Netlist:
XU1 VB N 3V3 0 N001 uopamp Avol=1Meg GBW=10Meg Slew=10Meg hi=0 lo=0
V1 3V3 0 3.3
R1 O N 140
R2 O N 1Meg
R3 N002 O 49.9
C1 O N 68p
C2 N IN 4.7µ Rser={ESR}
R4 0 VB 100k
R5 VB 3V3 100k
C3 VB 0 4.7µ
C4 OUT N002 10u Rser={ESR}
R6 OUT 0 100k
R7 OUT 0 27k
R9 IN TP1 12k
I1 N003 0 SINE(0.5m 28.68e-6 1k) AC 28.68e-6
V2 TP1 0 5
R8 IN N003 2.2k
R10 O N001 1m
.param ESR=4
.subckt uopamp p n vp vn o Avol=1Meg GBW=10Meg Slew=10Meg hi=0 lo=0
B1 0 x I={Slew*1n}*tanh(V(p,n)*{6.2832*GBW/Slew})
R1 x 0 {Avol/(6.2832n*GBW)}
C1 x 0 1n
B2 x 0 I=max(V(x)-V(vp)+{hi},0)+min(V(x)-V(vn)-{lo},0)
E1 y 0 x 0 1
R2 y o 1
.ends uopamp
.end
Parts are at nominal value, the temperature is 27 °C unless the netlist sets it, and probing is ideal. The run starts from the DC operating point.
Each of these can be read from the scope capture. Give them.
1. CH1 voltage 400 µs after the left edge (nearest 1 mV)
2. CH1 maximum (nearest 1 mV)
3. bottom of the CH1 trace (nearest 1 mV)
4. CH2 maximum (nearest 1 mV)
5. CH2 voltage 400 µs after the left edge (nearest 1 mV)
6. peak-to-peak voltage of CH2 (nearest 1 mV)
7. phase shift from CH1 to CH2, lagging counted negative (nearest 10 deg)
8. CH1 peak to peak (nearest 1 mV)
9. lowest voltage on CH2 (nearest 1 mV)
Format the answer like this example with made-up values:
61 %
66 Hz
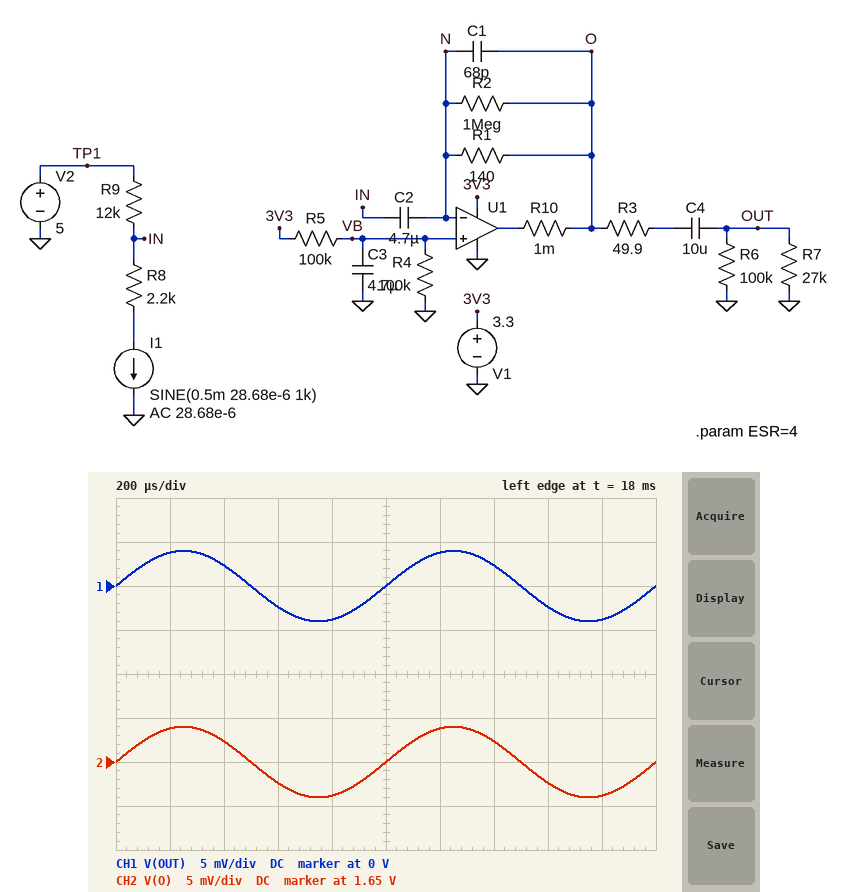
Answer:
2 mV
4 mV
-4 mV
1.654 V
1.652 V
8 mV
0 deg
8 mV
1.646 V
